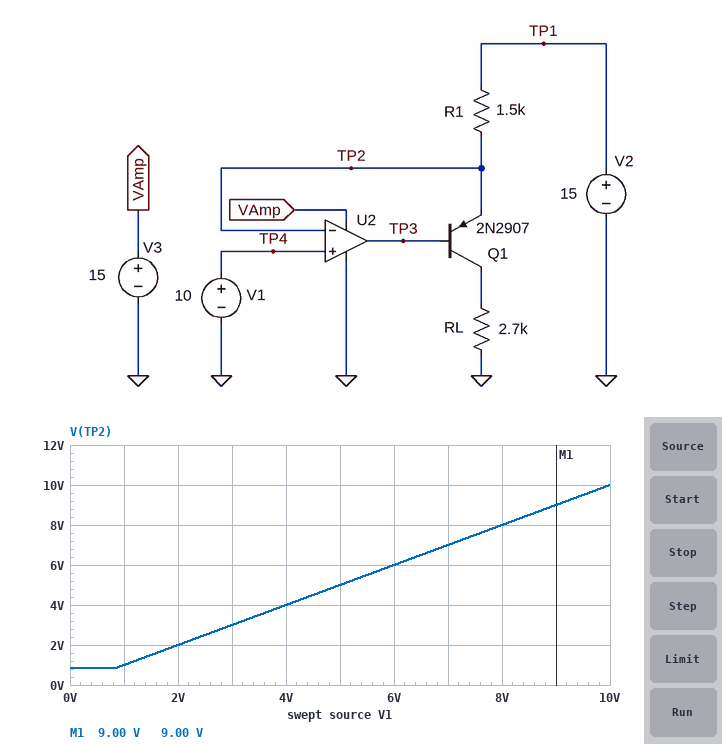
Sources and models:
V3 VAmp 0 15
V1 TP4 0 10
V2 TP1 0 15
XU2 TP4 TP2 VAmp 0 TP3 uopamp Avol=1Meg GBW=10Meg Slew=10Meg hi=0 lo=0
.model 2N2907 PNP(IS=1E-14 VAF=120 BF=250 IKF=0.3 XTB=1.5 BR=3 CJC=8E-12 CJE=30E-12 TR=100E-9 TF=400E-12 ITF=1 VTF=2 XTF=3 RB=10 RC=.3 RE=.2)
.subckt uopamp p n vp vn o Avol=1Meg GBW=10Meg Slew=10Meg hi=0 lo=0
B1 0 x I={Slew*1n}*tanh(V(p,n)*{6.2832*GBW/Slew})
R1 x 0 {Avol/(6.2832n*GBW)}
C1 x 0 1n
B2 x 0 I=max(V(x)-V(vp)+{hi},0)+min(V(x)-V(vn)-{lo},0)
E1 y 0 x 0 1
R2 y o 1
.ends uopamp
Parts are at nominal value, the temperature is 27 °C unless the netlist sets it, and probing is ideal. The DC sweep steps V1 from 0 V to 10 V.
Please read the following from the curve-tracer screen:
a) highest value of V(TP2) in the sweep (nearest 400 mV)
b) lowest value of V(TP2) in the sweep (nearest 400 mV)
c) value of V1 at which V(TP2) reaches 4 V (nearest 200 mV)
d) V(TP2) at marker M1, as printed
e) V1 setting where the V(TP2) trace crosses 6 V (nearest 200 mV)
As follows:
10.0 V
800 mV
4.0 V
9.00 V
6.0 V
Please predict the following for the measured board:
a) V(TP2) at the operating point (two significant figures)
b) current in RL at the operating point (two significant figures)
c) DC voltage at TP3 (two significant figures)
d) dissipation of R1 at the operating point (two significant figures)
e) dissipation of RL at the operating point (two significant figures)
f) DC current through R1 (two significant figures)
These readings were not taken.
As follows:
10 V
3.3 mA
9.3 V
17 mW
30 mW
3.3 mA
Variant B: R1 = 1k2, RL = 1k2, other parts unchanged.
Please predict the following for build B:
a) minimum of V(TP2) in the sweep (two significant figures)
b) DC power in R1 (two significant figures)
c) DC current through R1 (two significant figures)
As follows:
870 mV
21 mW
4.2 mA
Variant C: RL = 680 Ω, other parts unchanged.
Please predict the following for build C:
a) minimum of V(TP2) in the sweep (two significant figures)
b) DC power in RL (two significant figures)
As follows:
830 mV
7.5 mW
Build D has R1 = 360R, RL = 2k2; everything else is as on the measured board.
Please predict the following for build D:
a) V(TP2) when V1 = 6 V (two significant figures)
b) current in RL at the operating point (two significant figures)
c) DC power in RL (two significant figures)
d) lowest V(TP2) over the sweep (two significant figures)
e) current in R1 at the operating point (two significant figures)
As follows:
6.0 V
4.5 mA
45 mW
1.2 V
14 mA
